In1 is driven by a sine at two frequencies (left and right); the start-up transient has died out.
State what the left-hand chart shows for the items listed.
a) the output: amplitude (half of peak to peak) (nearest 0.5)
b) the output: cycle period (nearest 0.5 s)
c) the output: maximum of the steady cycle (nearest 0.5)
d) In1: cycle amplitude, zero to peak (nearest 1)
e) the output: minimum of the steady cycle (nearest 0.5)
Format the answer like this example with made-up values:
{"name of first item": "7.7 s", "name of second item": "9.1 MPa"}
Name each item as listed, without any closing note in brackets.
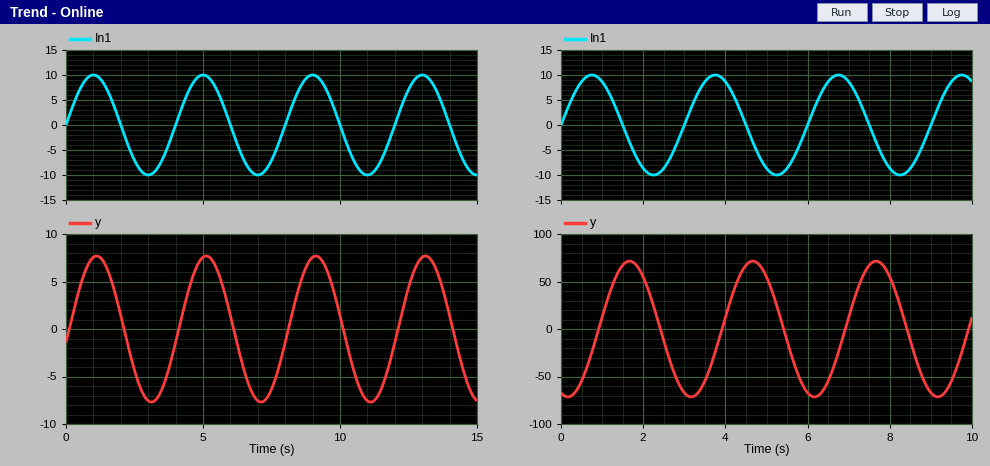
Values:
{"the output: amplitude (half of peak to peak)": "7.5", "the output: cycle period": "4.0 s", "the output: maximum of the steady cycle": "7.5", "In1: cycle amplitude, zero to peak": "10", "the output: minimum of the steady cycle": "-7.5"}
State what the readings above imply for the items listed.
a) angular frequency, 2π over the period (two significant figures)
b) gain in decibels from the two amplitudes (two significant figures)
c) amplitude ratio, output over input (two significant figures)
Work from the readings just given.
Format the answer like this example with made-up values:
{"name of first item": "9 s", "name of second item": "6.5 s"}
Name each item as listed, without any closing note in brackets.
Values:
{"angular frequency, 2π over the period": "1.6 rad/s", "gain in decibels from the two amplitudes": "-2.5 dB", "amplitude ratio, output over input": "0.75"}
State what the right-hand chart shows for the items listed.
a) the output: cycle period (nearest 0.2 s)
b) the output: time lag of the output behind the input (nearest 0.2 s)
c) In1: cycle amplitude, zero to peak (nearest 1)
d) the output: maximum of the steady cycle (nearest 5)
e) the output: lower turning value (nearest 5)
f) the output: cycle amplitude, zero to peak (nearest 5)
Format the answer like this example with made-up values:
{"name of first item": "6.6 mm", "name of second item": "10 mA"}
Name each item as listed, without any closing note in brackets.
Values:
{"the output: cycle period": "3.0 s", "the output: time lag of the output behind the input": "1.0 s", "In1: cycle amplitude, zero to peak": "10", "the output: maximum of the steady cycle": "70", "the output: lower turning value": "-70", "the output: cycle amplitude, zero to peak": "70"}
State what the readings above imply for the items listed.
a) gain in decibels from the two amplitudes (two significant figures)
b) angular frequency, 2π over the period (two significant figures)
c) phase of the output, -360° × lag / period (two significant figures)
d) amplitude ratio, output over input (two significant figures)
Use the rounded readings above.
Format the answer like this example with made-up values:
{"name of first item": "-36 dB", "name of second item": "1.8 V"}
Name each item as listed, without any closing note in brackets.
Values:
{"gain in decibels from the two amplitudes": "17 dB", "angular frequency, 2π over the period": "2.1 rad/s", "phase of the output, -360° × lag / period": "-120°", "amplitude ratio, output over input": "7.0"}
